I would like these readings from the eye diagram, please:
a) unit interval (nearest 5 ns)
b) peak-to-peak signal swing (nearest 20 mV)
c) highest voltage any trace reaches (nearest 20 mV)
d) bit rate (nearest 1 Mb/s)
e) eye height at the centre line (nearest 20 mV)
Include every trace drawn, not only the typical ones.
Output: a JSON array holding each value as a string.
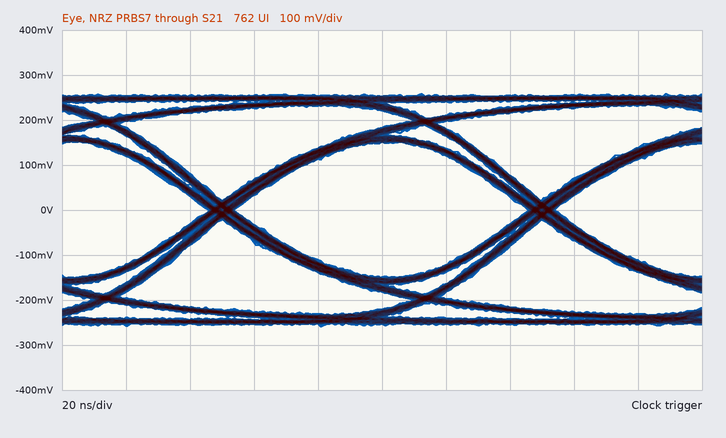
["100 ns", "520 mV", "260 mV", "10 Mb/s", "300 mV"]
